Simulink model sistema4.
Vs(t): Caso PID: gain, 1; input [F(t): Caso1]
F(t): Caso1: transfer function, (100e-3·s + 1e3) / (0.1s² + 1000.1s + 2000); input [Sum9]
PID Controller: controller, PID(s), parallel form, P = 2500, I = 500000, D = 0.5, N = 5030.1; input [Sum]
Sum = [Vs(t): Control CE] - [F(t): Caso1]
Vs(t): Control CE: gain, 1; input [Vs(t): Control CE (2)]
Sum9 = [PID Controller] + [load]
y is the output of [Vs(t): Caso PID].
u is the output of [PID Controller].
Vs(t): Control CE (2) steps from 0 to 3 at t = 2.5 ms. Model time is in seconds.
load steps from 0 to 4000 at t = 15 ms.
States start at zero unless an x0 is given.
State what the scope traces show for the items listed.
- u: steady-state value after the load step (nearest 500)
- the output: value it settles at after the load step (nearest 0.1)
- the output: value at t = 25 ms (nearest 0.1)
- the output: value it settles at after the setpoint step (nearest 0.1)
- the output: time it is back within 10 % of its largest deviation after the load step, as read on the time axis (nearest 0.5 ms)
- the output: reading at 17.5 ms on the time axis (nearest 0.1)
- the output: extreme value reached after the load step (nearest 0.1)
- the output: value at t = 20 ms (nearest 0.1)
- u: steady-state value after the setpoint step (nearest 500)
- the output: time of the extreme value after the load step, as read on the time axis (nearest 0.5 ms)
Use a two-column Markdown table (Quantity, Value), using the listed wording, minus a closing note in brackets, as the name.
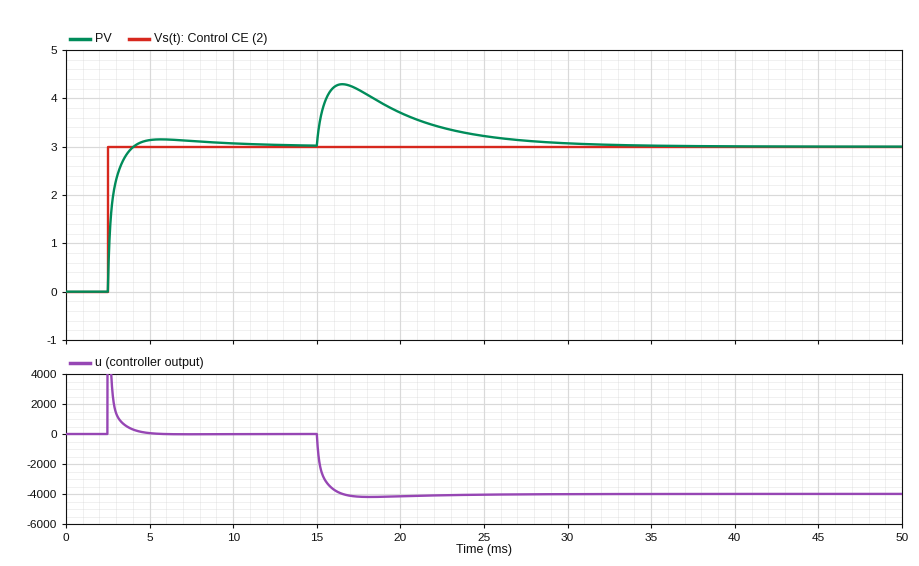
| Quantity | Value |
|---|---|
| u: steady-state value after the load step | -4000 |
| the output: value it settles at after the load step | 3.0 |
| the output: value at t = 25 ms | 3.2 |
| the output: value it settles at after the setpoint step | 3.0 |
| the output: time it is back within 10 % of its largest deviation after the load step, as read on the time axis | 27.5 ms |
| the output: reading at 17.5 ms on the time axis | 4.2 |
| the output: extreme value reached after the load step | 4.3 |
| the output: value at t = 20 ms | 3.7 |
| u: steady-state value after the setpoint step | 0 |
| the output: time of the extreme value after the load step, as read on the time axis | 16.5 ms |
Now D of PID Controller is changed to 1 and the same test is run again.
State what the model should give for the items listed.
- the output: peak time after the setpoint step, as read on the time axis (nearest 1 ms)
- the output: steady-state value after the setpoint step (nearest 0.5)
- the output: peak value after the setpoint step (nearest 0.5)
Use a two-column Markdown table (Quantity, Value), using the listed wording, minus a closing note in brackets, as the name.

| Quantity | Value |
|---|---|
| the output: peak time after the setpoint step, as read on the time axis | 6 ms |
| the output: steady-state value after the setpoint step | 3.0 |
| the output: peak value after the setpoint step | 3.0 |
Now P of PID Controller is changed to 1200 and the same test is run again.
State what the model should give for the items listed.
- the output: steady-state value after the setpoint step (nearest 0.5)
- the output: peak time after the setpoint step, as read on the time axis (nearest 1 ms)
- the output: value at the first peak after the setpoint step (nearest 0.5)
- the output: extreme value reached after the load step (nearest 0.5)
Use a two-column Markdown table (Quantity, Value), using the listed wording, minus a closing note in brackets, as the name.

| Quantity | Value |
|---|---|
| the output: steady-state value after the setpoint step | 3.0 |
| the output: peak time after the setpoint step, as read on the time axis | 6 ms |
| the output: value at the first peak after the setpoint step | 3.5 |
| the output: extreme value reached after the load step | 5.0 |
